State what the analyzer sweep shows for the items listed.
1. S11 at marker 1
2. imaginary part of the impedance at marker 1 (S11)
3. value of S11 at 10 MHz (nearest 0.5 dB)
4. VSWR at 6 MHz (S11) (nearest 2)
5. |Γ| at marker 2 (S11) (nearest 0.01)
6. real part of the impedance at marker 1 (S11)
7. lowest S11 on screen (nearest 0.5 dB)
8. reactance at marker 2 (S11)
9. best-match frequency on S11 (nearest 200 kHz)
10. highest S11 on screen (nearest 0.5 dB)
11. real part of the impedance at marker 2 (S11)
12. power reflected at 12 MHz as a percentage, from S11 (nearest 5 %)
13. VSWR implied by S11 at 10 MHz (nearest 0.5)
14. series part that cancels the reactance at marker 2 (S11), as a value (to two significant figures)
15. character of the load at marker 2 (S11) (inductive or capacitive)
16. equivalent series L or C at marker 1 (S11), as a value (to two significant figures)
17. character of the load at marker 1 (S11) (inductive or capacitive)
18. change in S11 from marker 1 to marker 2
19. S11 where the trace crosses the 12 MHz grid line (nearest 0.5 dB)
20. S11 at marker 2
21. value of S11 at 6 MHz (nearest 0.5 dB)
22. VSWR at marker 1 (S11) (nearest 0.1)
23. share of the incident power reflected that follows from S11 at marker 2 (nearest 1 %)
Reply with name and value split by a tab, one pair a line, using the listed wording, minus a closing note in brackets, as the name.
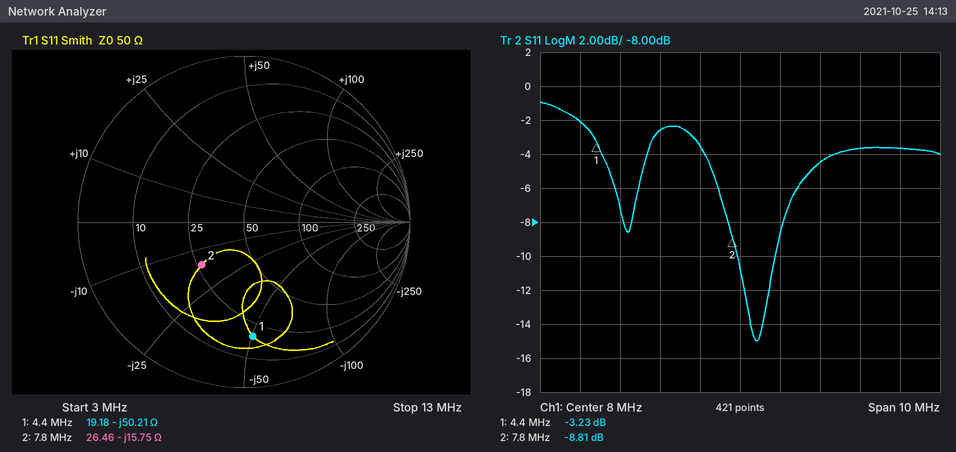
S11 at marker 1	-3.23 dB
imaginary part of the impedance at marker 1	-50.21 Ω
value of S11 at 10 MHz	-4.5 dB
VSWR at 6 MHz (S11)	6
|Γ| at marker 2 (S11)	0.36
real part of the impedance at marker 1	19.18 Ω
lowest S11 on screen	-15.0 dB
reactance at marker 2	-15.75 Ω
best-match frequency on S11	8.4 MHz
highest S11 on screen	-1.0 dB
real part of the impedance at marker 2	26.46 Ω
power reflected at 12 MHz as a percentage, from S11	45 %
VSWR implied by S11 at 10 MHz	4.0
series part that cancels the reactance at marker 2 (S11), as a value	320 nH
character of the load at marker 2 (S11)	capacitive
equivalent series L or C at marker 1 (S11), as a value	720 pF
character of the load at marker 1 (S11)	capacitive
change in S11 from marker 1 to marker 2	-5.58 dB
S11 where the trace crosses the 12 MHz grid line	-3.5 dB
S11 at marker 2	-8.81 dB
value of S11 at 6 MHz	-2.5 dB
VSWR at marker 1 (S11)	5.4
share of the incident power reflected that follows from S11 at marker 2	13 %
